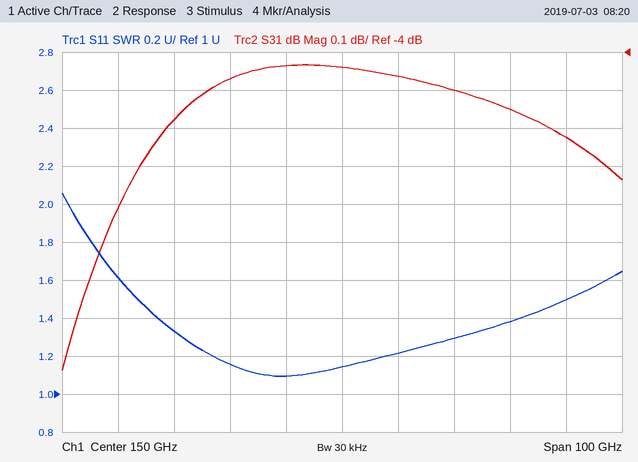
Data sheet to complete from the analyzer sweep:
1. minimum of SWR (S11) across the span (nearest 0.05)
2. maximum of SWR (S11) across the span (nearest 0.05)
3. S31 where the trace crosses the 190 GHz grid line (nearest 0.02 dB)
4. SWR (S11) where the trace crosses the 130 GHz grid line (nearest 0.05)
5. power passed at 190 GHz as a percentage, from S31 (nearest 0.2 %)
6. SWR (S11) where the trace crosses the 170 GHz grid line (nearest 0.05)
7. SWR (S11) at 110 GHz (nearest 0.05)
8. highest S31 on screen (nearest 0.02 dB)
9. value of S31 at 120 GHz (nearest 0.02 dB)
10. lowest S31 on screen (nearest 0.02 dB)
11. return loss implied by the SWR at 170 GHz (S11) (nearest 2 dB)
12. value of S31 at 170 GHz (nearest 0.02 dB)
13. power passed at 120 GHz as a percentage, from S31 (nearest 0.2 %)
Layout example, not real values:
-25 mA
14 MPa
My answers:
1.10
2.05
-4.22 dB
1.15
37.8 %
1.30
1.60
-4.04 dB
-4.18 dB
-4.84 dB
18 dB
-4.10 dB
38.2 %
